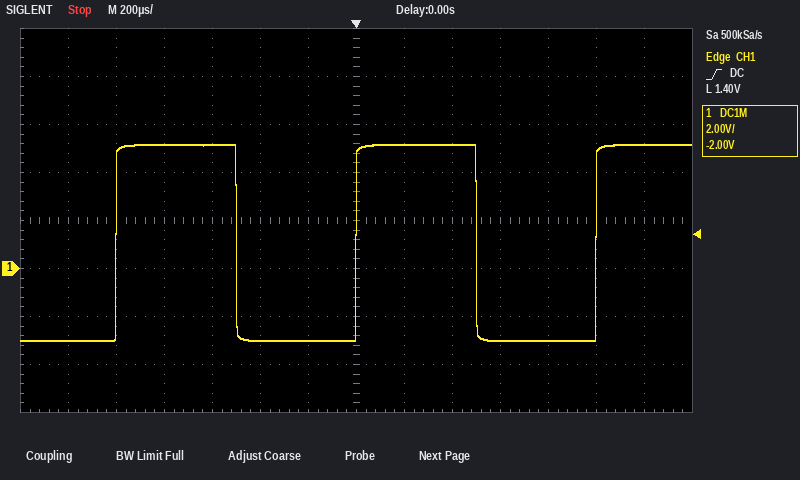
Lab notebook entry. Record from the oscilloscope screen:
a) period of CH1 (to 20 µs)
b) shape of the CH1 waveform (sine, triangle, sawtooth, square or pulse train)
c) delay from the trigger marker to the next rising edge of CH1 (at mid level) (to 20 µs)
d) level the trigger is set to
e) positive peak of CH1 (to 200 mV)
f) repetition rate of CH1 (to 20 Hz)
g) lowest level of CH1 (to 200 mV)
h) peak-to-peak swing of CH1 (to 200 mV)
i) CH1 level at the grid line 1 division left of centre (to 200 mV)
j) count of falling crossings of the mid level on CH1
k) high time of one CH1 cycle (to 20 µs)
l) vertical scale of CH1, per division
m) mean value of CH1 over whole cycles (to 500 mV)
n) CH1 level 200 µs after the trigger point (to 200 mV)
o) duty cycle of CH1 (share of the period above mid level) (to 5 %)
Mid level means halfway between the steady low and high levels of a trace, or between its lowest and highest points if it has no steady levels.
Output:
1.00 ms
square
1.00 ms
1.40 V
5.2 V
1.00 kHz
-3.0 V
8.2 V
-3.0 V
2
500 µs
2 V
1.0 V
5.2 V
50 %
